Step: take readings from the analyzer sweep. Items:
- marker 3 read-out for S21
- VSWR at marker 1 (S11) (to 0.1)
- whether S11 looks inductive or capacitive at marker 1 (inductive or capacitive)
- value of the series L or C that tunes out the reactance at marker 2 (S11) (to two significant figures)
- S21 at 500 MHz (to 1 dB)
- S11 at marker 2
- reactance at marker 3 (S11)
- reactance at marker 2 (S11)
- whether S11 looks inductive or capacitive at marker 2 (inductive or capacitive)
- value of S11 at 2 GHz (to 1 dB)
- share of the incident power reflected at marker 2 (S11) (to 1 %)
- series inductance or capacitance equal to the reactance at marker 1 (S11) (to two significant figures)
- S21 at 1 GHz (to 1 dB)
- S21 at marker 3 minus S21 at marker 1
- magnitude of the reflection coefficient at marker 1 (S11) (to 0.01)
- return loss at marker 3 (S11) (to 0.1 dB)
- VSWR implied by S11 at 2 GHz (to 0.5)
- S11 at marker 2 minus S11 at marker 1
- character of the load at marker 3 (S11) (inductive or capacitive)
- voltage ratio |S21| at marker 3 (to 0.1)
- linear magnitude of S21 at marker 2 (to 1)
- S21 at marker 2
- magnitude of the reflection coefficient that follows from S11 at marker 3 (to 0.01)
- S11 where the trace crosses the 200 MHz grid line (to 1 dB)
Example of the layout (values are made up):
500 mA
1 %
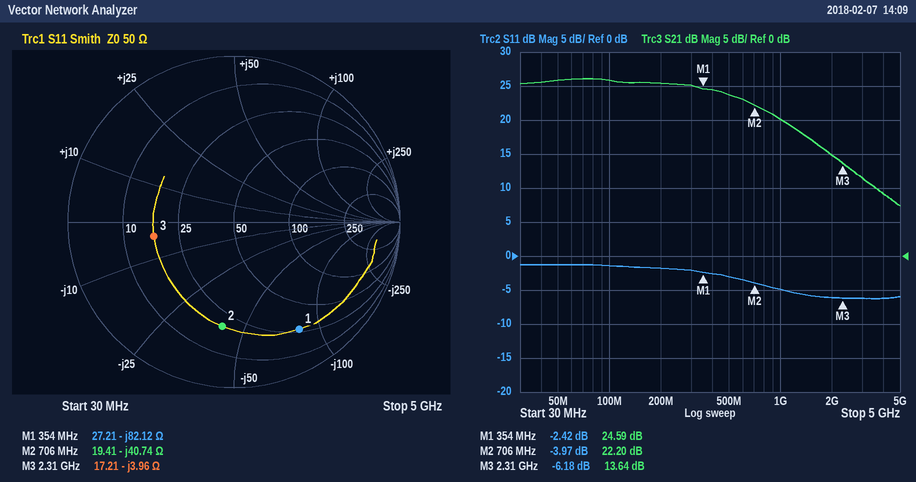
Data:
13.64 dB
7.2
capacitive
9.2 nH
24 dB
-3.97 dB
-3.96 Ω
-40.74 Ω
capacitive
-6 dB
40 %
5.5 pF
20 dB
-10.95 dB
0.76
6.2 dB
3.0
-1.55 dB
capacitive
4.8
13
22.20 dB
0.49
-2 dB
